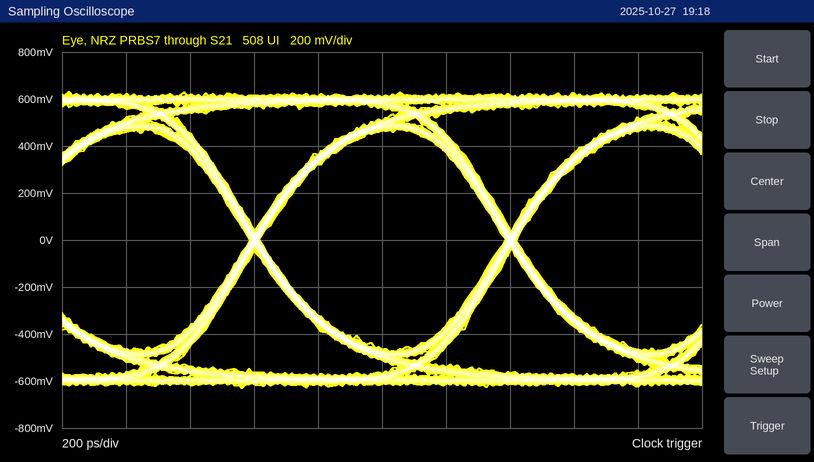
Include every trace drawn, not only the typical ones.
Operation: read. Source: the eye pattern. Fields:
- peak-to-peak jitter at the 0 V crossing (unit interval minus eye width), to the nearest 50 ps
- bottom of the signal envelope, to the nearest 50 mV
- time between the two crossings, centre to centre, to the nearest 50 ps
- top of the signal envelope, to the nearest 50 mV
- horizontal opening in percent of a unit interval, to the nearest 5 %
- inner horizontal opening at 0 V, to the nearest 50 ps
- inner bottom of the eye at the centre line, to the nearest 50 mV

50 ps
-650 mV
800 ps
650 mV
95 %
750 ps
-450 mV
